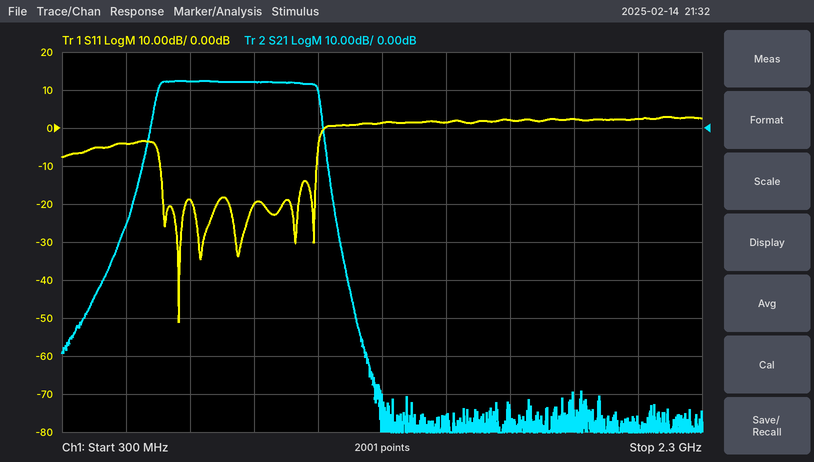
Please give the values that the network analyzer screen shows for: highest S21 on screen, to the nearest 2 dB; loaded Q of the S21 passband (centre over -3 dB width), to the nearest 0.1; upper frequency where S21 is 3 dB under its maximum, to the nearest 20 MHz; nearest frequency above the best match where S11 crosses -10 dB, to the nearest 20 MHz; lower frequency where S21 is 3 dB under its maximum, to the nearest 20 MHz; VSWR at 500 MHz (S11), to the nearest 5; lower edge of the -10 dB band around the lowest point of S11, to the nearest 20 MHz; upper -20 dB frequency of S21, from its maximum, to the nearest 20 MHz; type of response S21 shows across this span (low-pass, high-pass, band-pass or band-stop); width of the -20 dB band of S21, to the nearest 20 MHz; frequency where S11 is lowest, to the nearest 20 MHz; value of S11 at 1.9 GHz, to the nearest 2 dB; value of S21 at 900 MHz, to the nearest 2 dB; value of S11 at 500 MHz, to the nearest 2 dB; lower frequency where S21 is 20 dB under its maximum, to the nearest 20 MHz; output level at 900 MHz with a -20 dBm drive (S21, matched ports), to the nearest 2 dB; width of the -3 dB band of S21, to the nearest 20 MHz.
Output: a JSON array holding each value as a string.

["12 dB", "1.7", "1.10 GHz", "1.10 GHz", "600 MHz", "5", "600 MHz", "1.12 GHz", "band-pass", "560 MHz", "660 MHz", "2 dB", "12 dB", "-4 dB", "560 MHz", "-8 dBm", "500 MHz"]
